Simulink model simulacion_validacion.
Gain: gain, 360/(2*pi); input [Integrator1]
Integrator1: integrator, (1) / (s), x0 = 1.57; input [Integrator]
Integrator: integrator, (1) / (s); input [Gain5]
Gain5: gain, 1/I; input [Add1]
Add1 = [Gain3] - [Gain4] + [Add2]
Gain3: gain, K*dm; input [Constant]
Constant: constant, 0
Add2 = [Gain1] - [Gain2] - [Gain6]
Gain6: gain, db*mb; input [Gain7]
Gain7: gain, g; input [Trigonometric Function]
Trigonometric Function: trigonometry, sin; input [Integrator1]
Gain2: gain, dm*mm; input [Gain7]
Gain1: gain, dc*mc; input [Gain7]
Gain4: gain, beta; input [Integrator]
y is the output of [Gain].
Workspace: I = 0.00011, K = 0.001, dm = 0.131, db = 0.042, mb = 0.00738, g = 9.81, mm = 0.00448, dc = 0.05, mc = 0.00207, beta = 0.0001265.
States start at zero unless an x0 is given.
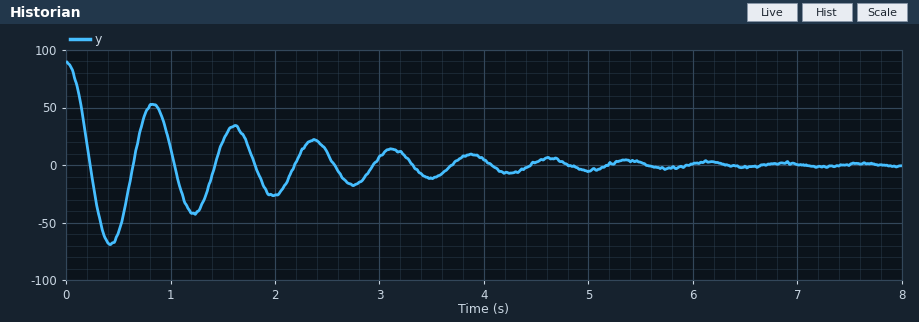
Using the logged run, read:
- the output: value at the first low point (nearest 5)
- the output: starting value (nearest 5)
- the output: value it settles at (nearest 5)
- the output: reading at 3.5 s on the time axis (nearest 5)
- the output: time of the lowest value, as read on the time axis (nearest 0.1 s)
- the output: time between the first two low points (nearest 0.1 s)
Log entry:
-70
90
0
-10
0.4 s
0.8 s
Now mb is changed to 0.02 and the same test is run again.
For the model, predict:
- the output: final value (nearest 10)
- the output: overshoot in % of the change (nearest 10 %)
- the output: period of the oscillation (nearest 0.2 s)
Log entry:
0
80 %
0.6 s
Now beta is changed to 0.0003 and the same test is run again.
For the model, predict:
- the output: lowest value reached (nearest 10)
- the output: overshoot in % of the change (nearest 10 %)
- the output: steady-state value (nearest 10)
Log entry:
-50
50 %
0
